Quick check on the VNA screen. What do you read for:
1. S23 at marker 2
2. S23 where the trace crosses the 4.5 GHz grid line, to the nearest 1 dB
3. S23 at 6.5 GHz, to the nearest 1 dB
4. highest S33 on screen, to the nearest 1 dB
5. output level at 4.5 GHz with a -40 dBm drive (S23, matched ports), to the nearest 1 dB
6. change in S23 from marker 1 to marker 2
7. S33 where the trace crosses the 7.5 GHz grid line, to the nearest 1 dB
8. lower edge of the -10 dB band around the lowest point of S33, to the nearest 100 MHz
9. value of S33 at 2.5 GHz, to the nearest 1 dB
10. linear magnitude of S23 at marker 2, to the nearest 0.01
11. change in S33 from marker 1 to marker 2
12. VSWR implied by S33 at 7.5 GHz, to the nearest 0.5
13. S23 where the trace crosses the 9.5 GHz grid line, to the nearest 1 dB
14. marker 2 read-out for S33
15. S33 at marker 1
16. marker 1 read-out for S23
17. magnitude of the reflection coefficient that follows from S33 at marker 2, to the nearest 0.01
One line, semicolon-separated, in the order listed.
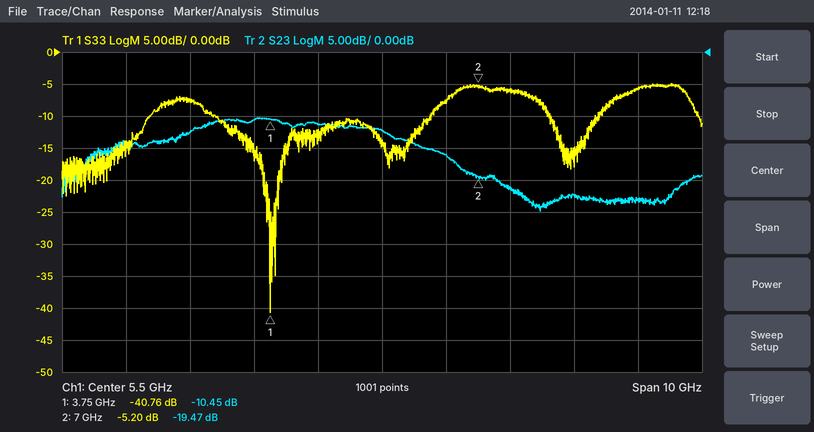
-19.47 dB; -11 dB; -16 dB; -5 dB; -51 dBm; -9.02 dB; -6 dB; 2.9 GHz; -8 dB; 0.11; 35.56 dB; 3.0; -23 dB; -5.20 dB; -40.76 dB; -10.45 dB; 0.55
